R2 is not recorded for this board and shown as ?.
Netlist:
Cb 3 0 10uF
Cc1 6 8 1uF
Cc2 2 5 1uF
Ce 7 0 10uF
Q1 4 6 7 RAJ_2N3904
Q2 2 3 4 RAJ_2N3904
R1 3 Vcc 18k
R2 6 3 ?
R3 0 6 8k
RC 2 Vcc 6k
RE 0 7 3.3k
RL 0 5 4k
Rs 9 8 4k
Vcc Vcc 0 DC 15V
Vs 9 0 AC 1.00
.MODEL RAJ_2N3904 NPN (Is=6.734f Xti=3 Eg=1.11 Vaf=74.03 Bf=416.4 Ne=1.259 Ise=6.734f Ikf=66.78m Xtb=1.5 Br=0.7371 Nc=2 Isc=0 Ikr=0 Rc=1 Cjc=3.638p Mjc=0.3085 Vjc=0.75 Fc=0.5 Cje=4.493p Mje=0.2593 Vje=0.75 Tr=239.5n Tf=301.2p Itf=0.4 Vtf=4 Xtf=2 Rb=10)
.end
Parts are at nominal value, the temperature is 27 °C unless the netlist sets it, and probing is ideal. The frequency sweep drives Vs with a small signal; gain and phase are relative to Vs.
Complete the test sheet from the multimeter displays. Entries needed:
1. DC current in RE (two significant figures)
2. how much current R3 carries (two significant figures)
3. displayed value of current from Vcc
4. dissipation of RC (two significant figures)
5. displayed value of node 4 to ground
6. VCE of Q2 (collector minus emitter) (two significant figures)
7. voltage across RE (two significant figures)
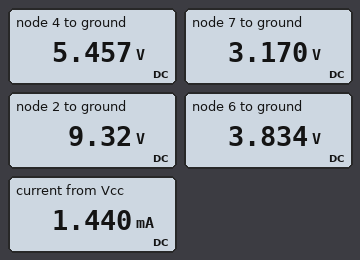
960 µA
480 µA
1.440 mA
5.4 mW
5.457 V
3.9 V
3.2 V
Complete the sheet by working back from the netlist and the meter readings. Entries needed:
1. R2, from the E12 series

4.7 kΩ
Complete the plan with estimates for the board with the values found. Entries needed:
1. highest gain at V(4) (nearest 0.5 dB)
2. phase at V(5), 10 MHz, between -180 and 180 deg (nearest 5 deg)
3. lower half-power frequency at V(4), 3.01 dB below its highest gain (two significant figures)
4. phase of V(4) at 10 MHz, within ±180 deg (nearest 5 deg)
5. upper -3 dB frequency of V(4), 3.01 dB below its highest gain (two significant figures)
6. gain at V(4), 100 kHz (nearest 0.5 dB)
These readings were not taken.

-10.0 dB
100 deg
420 Hz
125 deg
5.9 MHz
-10.0 dB
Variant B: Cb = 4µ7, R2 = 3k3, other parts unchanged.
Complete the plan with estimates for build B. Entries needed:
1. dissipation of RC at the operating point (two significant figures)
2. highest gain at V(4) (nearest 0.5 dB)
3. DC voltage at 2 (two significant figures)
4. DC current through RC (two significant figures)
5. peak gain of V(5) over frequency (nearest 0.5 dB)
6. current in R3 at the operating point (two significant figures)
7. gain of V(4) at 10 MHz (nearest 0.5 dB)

6.0 mW
-11.0 dB
9.0 V
1.0 mA
28.0 dB
500 µA
-16.5 dB
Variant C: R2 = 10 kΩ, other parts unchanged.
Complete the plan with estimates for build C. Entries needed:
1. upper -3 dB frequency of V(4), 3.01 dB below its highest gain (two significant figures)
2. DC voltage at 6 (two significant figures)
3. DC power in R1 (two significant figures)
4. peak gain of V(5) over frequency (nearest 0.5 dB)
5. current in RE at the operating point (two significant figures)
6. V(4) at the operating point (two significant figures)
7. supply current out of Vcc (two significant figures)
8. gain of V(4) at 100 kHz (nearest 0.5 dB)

5.5 MHz
3.3 V
3.2 mW
28.5 dB
790 µA
6.8 V
1.2 mA
-8.5 dB
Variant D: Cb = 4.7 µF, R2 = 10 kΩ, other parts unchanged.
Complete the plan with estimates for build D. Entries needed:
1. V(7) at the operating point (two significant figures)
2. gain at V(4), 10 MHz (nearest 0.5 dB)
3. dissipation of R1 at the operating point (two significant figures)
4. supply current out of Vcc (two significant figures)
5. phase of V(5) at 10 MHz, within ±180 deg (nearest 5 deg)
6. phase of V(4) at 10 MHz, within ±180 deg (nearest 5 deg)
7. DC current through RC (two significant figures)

2.6 V
-14.5 dB
3.2 mW
1.2 mA
95 deg
120 deg
780 µA
